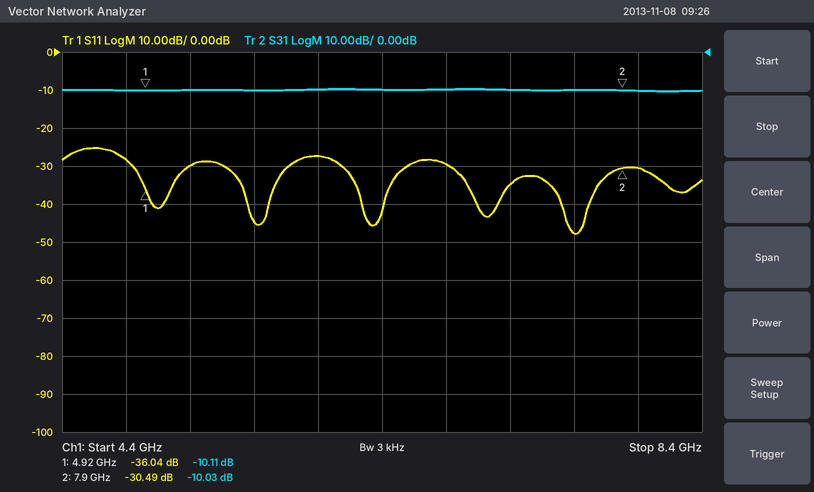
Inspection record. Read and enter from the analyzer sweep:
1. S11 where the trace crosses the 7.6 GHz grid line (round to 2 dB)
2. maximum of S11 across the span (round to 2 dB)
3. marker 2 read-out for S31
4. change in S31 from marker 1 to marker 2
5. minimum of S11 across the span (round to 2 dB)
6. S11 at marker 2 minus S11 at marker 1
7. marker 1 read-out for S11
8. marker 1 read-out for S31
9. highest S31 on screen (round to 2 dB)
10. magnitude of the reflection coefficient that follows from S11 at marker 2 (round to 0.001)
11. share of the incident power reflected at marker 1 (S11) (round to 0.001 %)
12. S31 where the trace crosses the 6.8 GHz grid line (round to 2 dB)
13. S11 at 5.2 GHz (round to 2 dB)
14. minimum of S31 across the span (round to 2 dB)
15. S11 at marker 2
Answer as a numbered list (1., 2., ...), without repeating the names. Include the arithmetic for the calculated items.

1. -48 dB
2. -26 dB
3. -10.03 dB
4. -10.03 − (-10.11) = 0.08 dB
5. -48 dB
6. -30.49 − (-36.04) = 5.55 dB
7. -36.04 dB
8. -10.11 dB
9. -10 dB
10. 10^(-30.49/20) ≈ 0.030
11. 10^(-36.04/10) ≈ 0.025 %
12. -10 dB
13. -30 dB
14. -10 dB
15. -30.49 dB
